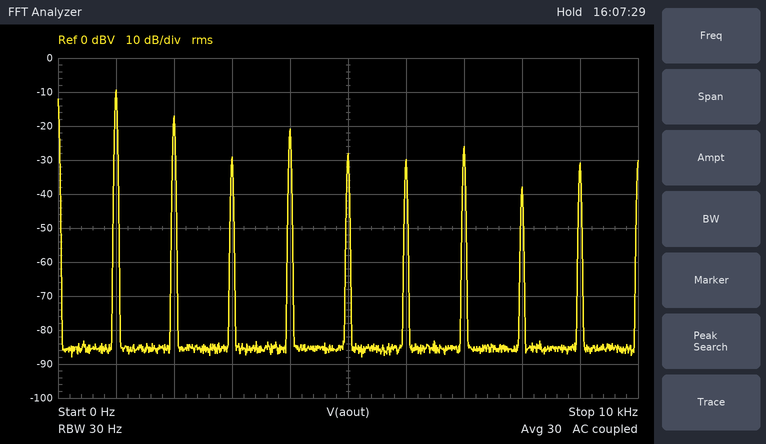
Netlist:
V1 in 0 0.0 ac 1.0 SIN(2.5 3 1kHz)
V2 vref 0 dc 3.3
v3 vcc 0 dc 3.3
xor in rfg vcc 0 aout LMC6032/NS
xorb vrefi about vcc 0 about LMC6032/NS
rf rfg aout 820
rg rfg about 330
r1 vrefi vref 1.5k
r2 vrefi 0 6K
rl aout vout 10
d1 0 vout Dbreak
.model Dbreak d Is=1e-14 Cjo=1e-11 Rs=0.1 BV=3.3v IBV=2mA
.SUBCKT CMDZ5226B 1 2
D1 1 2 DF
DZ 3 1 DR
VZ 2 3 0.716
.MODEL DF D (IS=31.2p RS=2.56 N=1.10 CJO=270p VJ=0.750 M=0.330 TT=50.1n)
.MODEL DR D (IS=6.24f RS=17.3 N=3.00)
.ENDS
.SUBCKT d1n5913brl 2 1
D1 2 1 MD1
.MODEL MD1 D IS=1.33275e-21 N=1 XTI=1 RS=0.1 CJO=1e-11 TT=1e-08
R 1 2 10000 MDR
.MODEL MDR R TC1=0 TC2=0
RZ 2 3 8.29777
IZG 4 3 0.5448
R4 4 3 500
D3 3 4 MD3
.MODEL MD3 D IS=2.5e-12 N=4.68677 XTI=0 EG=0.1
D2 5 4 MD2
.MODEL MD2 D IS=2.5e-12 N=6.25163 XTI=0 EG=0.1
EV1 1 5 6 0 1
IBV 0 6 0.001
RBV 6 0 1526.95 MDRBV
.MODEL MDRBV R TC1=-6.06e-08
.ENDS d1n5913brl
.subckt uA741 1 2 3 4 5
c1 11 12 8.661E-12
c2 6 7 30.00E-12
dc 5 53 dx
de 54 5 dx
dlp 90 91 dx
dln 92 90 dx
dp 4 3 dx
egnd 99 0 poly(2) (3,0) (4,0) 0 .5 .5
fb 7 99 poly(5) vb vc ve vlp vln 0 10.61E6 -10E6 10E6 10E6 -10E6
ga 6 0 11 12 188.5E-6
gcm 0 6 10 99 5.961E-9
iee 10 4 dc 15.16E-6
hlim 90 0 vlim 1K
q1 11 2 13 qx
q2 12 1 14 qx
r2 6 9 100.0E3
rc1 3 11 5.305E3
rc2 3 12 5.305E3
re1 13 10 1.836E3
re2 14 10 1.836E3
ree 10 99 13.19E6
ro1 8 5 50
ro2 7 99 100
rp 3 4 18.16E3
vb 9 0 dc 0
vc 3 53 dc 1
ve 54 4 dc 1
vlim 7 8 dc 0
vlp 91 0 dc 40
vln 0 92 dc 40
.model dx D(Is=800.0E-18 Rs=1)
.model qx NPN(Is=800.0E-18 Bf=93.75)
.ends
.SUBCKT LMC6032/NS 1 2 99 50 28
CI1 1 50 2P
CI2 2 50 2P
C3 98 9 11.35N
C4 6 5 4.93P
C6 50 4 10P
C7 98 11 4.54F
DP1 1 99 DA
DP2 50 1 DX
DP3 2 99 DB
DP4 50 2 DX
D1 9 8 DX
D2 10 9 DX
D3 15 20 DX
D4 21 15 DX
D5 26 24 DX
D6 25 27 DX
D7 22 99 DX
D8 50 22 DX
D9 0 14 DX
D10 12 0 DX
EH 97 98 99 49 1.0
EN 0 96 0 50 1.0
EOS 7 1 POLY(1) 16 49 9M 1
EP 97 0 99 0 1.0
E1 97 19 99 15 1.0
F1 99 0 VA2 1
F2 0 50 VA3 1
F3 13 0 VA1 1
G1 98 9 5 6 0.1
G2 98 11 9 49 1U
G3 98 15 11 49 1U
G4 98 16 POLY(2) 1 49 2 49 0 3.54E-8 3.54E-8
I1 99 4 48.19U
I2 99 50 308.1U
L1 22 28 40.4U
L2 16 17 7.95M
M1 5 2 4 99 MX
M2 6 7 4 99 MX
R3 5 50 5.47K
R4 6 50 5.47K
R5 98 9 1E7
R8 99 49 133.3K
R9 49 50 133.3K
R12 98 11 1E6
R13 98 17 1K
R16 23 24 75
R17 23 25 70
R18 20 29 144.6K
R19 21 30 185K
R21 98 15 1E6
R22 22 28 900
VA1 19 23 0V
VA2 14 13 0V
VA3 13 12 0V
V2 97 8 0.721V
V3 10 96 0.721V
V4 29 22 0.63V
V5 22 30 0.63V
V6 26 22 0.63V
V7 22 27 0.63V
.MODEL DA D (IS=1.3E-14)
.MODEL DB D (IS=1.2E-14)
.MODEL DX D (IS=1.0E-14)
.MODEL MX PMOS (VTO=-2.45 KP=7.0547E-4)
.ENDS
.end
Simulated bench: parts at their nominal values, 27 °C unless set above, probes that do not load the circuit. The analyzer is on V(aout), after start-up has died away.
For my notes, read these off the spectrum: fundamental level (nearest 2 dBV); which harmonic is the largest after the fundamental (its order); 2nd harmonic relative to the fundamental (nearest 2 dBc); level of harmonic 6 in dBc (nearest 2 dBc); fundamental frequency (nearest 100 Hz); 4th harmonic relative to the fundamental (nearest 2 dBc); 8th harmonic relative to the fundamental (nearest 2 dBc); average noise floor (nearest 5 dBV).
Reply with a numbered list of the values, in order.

1. -10 dBV
2. 2
3. -8 dBc
4. -20 dBc
5. 1.0 kHz
6. -12 dBc
7. -28 dBc
8. -85 dBV
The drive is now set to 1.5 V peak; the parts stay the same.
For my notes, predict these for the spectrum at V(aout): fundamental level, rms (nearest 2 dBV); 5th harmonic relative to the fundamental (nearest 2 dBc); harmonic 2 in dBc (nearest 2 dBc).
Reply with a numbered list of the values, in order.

1. -14 dBV
2. -24 dBc
3. -2 dBc
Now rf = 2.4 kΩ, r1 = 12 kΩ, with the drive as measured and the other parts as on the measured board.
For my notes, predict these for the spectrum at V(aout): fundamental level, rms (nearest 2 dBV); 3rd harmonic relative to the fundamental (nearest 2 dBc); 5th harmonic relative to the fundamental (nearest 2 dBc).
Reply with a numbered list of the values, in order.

1. 2 dBV
2. -24 dBc
3. -16 dBc
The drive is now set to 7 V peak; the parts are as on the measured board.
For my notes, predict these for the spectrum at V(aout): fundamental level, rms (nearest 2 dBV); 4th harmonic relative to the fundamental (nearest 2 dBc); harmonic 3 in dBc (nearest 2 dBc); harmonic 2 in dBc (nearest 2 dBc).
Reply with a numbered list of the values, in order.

1. -8 dBV
2. -16 dBc
3. -10 dBc
4. -16 dBc
